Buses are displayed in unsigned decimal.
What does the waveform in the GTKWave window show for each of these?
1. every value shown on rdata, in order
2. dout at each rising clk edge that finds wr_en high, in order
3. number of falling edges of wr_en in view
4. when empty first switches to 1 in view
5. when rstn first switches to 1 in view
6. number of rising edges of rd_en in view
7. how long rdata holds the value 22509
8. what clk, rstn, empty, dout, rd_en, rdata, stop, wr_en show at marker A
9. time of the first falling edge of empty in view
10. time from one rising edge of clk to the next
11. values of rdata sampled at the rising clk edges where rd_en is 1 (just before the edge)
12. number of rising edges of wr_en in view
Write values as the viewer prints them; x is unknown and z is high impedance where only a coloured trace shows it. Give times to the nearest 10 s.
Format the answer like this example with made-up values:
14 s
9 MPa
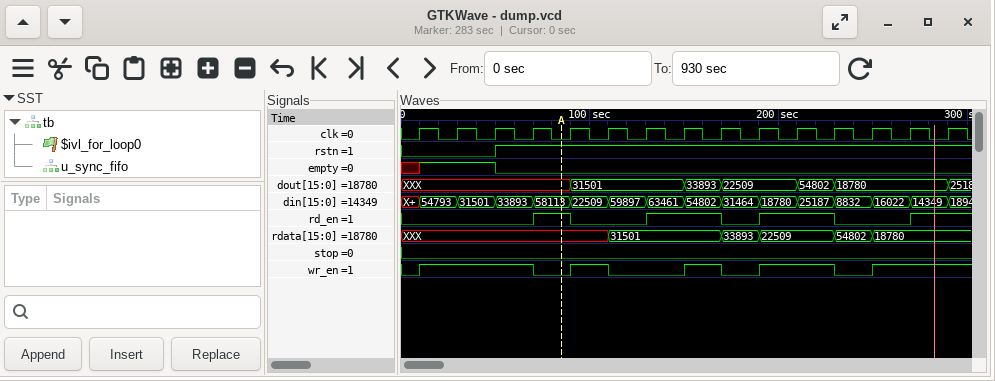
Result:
XXX, 31501, 33893, 22509, 54802, 18780
XXX, XXX, XXX, 31501, 33893, 22509, 54802, 18780, 18780
4
10 s
50 s
4
40 s
clk=0, rstn=1, empty=0, dout=XXX, rd_en=1, rdata=XXX, stop=0, wr_en=0
50 s
20 s
XXX, 31501, 31501, 22509, 22509, 18780
5
